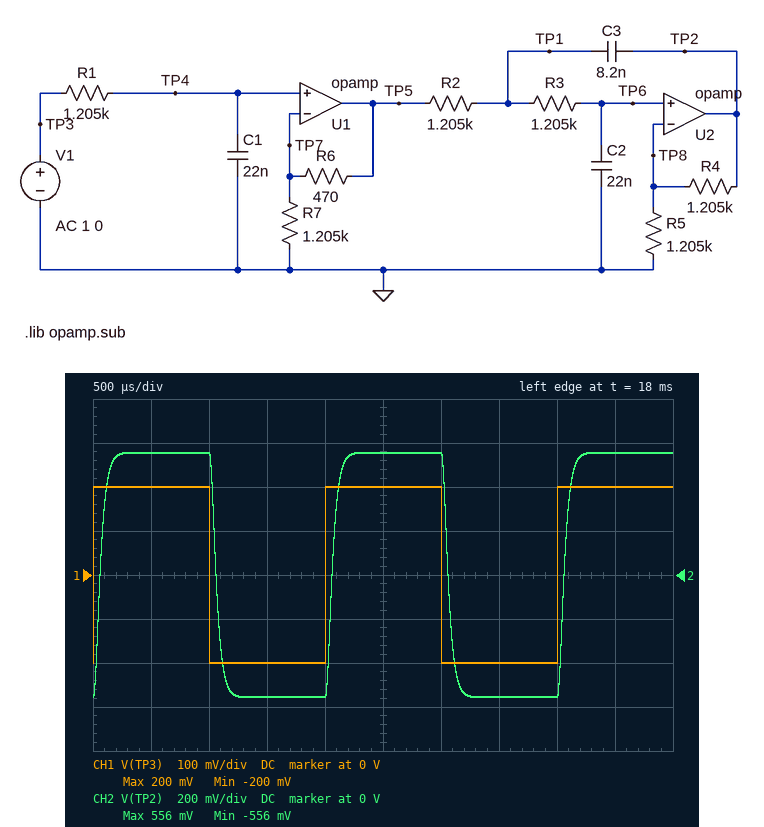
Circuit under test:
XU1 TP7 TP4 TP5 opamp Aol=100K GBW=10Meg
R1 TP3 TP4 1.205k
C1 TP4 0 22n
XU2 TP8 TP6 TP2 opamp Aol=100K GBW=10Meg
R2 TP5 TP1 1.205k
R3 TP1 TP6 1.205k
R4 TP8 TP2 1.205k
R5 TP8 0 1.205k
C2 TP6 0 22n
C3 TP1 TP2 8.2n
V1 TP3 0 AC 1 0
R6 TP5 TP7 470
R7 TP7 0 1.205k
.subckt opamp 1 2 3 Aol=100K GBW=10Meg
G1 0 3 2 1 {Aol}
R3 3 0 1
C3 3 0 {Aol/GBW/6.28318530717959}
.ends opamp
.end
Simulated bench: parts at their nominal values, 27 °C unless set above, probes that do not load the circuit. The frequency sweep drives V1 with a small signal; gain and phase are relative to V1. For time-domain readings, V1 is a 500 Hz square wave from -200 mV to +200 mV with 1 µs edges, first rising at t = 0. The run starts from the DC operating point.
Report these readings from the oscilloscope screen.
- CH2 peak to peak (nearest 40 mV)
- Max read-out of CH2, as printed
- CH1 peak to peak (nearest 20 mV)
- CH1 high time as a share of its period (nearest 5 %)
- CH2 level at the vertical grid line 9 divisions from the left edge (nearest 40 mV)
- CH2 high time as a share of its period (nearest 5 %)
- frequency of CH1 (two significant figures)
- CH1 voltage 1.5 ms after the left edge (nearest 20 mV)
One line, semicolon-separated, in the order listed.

1.12 V; 556 mV; 400 mV; 50 %; 560 mV; 50 %; 500 Hz; -200 mV
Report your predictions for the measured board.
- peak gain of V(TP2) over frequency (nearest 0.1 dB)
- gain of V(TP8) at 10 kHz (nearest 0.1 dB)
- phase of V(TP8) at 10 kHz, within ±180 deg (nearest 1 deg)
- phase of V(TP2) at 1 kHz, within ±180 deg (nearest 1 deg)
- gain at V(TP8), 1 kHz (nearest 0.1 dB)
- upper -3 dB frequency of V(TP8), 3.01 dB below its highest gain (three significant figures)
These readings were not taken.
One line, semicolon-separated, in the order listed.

8.9 dB; -11.6 dB; -150 deg; -25 deg; 2.5 dB; 3.21 kHz
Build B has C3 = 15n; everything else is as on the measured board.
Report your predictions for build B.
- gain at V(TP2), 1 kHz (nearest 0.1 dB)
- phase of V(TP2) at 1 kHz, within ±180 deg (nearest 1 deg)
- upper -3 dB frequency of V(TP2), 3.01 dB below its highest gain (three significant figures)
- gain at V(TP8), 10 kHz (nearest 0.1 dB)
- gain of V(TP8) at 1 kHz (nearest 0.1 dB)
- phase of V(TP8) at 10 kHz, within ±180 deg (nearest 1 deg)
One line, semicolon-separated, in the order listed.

8.7 dB; -22 deg; 4.32 kHz; -10.4 dB; 2.7 dB; -171 deg
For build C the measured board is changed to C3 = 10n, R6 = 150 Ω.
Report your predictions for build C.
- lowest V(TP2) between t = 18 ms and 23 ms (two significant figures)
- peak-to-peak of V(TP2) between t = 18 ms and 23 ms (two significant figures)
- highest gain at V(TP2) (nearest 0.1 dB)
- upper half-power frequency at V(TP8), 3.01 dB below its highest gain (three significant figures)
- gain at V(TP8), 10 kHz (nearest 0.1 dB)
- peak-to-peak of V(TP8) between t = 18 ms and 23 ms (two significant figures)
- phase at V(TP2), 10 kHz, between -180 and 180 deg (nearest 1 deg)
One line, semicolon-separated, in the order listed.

-450 mV; 900 mV; 7.0 dB; 3.44 kHz; -13.0 dB; 450 mV; -155 deg
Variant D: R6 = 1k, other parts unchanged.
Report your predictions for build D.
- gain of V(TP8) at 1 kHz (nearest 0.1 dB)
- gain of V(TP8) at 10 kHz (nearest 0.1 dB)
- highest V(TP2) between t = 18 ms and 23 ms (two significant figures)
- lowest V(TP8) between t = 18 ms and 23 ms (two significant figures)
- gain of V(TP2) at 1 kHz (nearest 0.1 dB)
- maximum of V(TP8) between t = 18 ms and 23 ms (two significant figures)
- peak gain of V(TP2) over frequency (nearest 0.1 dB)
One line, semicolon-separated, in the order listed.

4.9 dB; -9.2 dB; 730 mV; -370 mV; 10.9 dB; 370 mV; 11.3 dB
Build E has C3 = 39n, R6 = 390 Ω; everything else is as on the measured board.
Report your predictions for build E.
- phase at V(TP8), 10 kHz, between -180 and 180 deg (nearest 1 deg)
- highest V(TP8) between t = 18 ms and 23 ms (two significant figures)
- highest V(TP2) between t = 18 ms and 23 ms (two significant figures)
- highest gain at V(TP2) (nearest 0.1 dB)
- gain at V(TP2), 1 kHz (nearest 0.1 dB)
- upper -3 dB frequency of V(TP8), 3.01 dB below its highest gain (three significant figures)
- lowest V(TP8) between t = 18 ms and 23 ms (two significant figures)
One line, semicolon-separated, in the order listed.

126 deg; 610 mV; 1.2 V; 21.9 dB; 8.8 dB; 4.82 kHz; -610 mV
